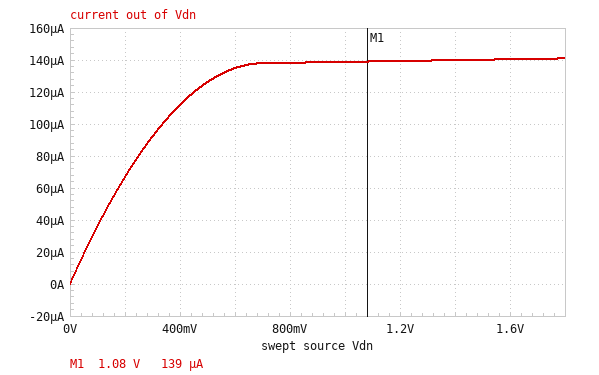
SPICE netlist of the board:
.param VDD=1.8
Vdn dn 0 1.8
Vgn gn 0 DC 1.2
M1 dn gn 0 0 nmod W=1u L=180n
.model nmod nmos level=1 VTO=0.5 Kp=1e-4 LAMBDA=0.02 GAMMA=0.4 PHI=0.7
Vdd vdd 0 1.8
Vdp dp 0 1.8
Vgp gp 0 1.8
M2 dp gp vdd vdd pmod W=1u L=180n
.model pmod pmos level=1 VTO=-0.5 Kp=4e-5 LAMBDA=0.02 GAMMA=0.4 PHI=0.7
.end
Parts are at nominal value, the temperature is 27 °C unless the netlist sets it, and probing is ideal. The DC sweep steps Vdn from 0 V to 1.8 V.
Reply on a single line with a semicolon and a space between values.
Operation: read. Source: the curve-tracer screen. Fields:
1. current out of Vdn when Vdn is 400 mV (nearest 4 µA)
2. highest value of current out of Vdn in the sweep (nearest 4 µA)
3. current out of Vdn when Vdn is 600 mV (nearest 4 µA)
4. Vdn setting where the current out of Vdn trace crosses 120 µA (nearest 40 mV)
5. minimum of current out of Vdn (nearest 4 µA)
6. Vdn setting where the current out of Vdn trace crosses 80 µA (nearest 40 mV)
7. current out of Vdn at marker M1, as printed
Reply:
112 µA; 140 µA; 136 µA; 440 mV; 0 A; 240 mV; 139 µA
